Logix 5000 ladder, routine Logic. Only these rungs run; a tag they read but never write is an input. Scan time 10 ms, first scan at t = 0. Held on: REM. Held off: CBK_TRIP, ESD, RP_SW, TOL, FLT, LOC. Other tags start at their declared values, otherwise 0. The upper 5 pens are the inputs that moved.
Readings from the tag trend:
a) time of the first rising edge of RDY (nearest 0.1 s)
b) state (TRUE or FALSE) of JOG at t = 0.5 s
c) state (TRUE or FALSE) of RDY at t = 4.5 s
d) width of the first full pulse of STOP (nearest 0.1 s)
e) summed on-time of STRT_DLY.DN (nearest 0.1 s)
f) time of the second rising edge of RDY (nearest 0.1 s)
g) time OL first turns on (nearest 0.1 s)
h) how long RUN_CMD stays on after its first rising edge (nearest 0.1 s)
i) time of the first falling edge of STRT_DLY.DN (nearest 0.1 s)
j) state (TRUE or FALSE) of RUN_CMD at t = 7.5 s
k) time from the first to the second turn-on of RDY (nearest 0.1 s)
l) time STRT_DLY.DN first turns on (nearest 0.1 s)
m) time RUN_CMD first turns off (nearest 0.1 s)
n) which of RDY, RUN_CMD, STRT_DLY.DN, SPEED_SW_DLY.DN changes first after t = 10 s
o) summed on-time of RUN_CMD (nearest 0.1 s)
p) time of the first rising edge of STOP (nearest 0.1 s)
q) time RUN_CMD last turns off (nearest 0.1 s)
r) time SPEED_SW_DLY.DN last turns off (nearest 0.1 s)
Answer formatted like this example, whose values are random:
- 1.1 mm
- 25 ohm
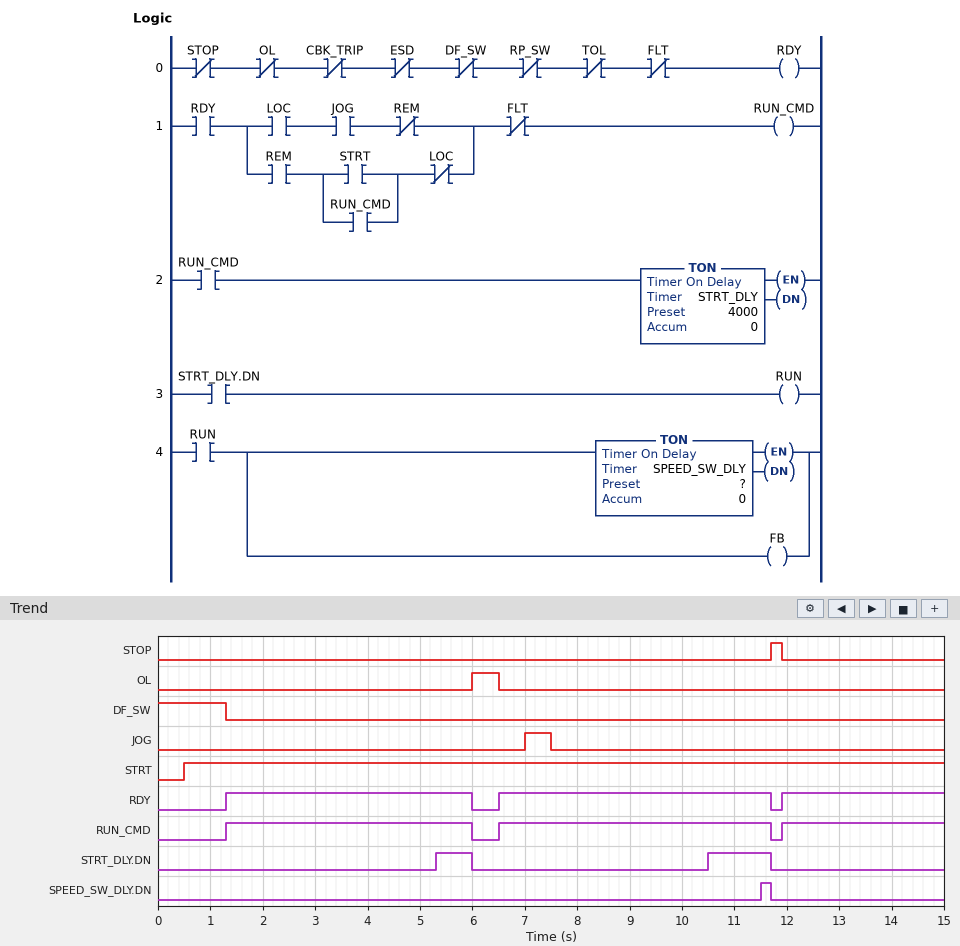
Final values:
- 1.3 s
- FALSE
- TRUE
- 0.2 s
- 1.9 s
- 6.5 s
- 6.0 s
- 4.7 s
- 6.0 s
- TRUE
- 5.2 s
- 5.3 s
- 6.0 s
- STRT_DLY.DN
- 13.0 s
- 11.7 s
- 11.7 s
- 11.7 s
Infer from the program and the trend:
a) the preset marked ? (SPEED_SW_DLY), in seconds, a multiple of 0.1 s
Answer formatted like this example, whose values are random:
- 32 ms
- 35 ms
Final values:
- 1.0 s
